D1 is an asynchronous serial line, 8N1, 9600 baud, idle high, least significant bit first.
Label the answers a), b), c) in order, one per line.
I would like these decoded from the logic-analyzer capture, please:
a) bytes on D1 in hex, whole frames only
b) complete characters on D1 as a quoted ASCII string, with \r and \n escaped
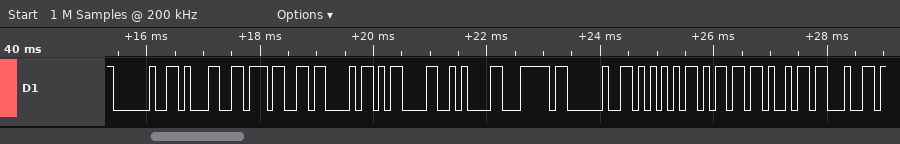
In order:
a) 20 31 37 43 0D 0A 7C 20 55 6D 69 64
b) " 17C\r\n| Umid"
